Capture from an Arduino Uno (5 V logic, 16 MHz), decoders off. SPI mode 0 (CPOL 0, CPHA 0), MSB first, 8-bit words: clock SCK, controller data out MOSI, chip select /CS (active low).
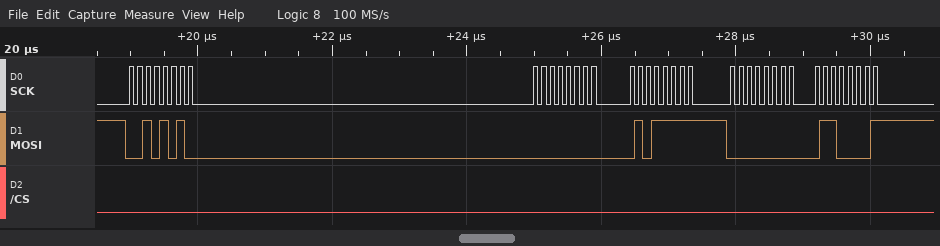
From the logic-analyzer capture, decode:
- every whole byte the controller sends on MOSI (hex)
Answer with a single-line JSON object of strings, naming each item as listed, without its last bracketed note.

{"every whole byte the controller sends on MOSI": "2A 00 5F 00 61"}
